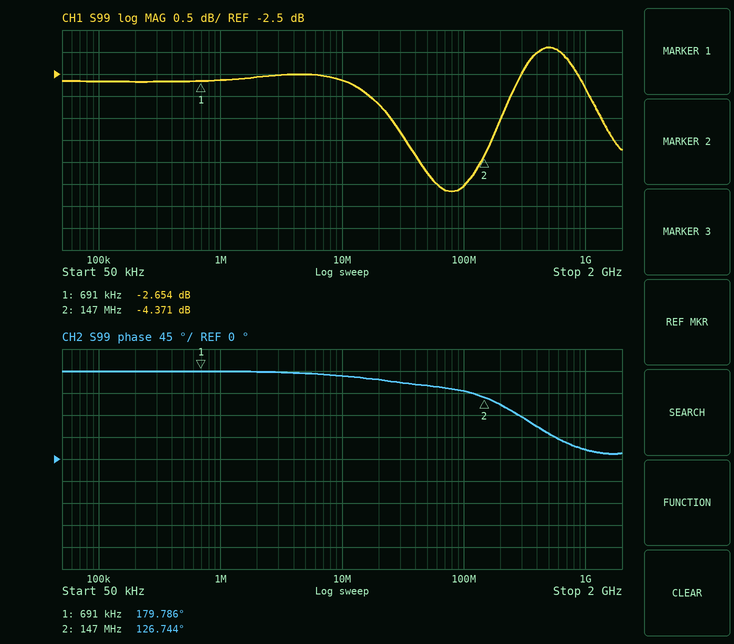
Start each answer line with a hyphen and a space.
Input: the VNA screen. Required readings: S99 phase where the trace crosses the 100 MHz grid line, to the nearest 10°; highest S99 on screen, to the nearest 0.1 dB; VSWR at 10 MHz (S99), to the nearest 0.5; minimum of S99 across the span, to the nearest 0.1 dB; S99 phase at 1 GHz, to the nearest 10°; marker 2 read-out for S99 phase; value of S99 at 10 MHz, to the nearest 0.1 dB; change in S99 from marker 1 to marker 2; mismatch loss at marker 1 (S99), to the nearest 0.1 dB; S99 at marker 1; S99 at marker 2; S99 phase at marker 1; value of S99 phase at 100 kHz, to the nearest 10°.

- 140°
- -1.9 dB
- 6.5
- -5.2 dB
- 20°
- 126.744°
- -2.6 dB
- -1.717 dB
- 3.4 dB
- -2.654 dB
- -4.371 dB
- 179.786°
- 180°
